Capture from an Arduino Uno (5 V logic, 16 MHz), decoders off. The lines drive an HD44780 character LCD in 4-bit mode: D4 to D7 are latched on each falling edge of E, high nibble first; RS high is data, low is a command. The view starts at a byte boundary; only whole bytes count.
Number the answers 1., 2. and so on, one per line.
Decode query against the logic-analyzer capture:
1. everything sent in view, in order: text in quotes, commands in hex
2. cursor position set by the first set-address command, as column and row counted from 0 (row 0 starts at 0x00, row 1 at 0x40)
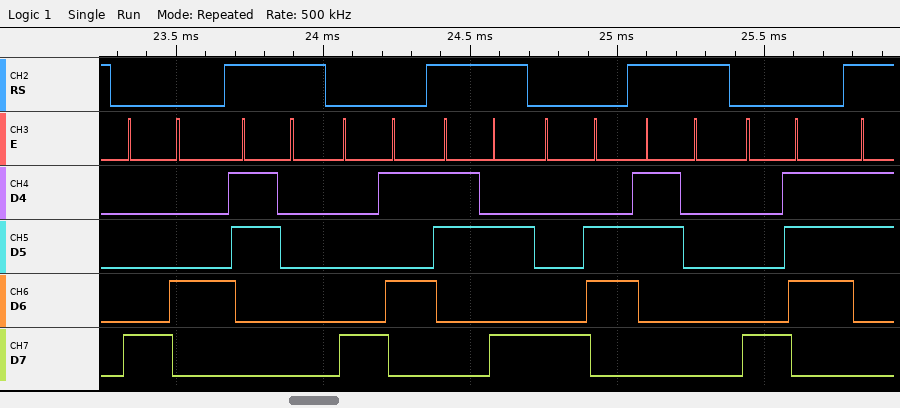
1. 0x84 "0" 0x85 ":" 0x86 "0" 0x87
2. column 4, row 0
